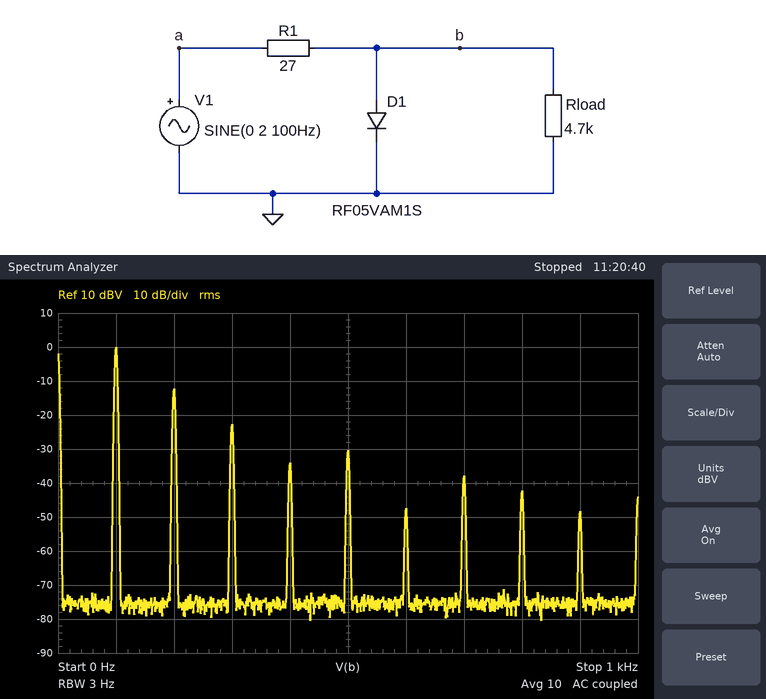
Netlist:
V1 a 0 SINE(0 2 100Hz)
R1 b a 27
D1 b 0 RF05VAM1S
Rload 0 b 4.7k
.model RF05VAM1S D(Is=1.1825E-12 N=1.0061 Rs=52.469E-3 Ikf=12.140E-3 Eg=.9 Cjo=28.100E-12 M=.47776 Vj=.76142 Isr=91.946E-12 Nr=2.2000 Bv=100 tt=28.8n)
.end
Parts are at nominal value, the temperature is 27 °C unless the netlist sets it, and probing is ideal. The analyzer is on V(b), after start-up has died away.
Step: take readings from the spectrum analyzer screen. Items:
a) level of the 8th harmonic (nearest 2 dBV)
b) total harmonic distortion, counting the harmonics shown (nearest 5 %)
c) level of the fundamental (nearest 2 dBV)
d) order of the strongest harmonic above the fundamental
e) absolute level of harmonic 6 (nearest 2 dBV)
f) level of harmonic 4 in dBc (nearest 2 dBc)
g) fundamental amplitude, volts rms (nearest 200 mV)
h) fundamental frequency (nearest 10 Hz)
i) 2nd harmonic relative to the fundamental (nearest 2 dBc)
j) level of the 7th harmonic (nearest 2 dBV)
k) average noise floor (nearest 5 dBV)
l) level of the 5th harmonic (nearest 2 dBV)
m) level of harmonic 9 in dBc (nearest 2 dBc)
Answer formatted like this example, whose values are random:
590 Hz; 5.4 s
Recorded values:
-42 dBV; 25 %; 0 dBV; 2; -48 dBV; -34 dBc; 1.0 V; 100 Hz; -12 dBc; -38 dBV; -75 dBV; -30 dBV; -48 dBc
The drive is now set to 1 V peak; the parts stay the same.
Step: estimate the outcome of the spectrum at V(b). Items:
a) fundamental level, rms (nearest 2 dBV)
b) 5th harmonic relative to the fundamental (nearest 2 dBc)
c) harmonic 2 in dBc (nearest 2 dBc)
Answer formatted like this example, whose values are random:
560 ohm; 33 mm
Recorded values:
-4 dBV; -48 dBc; -18 dBc
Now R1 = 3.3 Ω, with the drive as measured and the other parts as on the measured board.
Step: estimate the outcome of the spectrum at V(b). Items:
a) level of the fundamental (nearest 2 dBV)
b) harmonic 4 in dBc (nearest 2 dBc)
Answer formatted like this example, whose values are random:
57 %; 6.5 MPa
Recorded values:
0 dBV; -40 dBc
